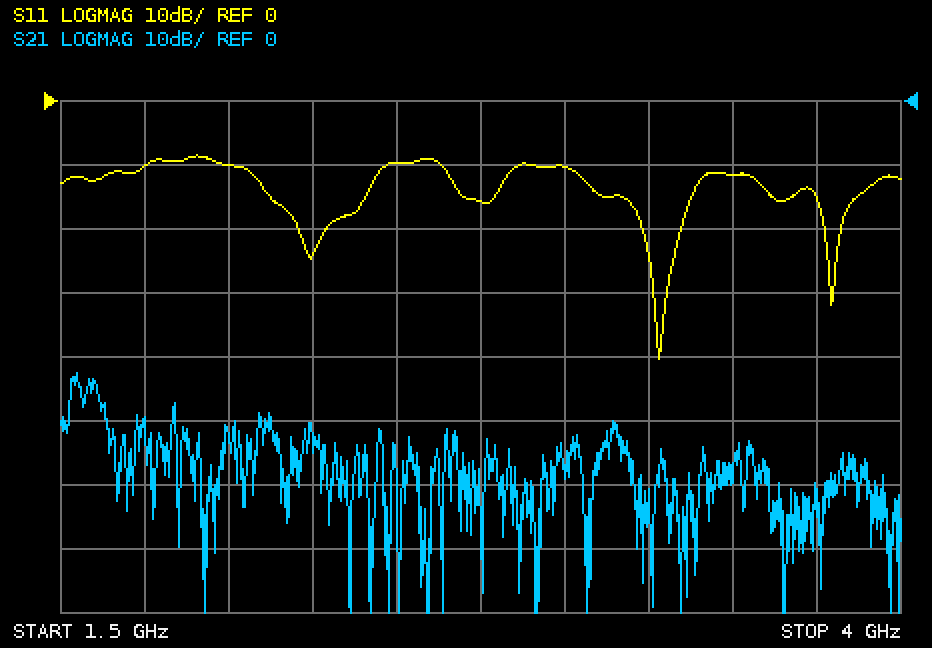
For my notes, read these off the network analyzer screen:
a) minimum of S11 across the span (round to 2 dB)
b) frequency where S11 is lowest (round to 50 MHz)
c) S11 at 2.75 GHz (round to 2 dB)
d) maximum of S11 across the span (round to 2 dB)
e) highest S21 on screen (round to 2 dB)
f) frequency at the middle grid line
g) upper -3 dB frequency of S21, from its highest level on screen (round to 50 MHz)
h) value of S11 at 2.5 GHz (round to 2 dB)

-40 dB
3.30 GHz
-16 dB
-8 dB
-42 dB
2.75 GHz
1.55 GHz
-10 dB
